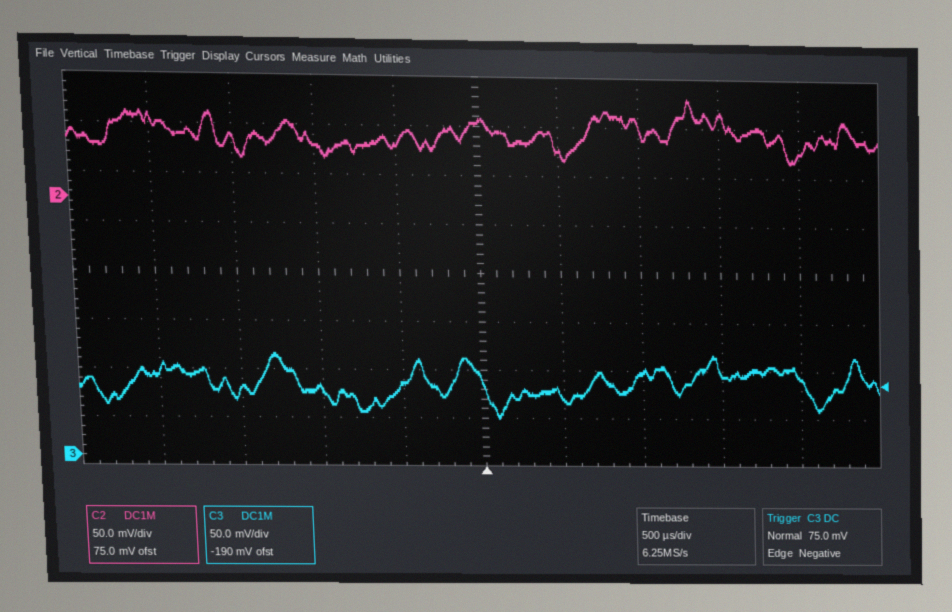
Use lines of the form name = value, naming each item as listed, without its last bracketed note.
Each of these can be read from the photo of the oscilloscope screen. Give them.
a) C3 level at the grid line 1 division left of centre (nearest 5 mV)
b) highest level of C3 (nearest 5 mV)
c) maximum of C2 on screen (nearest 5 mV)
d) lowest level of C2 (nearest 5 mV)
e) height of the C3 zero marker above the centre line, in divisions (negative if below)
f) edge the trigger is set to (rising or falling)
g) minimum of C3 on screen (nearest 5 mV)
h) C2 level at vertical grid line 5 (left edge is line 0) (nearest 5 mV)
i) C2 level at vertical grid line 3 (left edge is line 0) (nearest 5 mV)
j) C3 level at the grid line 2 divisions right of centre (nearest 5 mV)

C3 level at the grid line 1 division left of centre = 75 mV
highest level of C3 = 105 mV
maximum of C2 on screen = 105 mV
lowest level of C2 = 40 mV
height of the C3 zero marker above the centre line, in divisions = -3.8 div
edge the trigger is set to = falling
minimum of C3 on screen = 40 mV
C2 level at vertical grid line 5 (left edge is line 0) = 80 mV
C2 level at vertical grid line 3 (left edge is line 0) = 55 mV
C3 level at the grid line 2 divisions right of centre = 90 mV
